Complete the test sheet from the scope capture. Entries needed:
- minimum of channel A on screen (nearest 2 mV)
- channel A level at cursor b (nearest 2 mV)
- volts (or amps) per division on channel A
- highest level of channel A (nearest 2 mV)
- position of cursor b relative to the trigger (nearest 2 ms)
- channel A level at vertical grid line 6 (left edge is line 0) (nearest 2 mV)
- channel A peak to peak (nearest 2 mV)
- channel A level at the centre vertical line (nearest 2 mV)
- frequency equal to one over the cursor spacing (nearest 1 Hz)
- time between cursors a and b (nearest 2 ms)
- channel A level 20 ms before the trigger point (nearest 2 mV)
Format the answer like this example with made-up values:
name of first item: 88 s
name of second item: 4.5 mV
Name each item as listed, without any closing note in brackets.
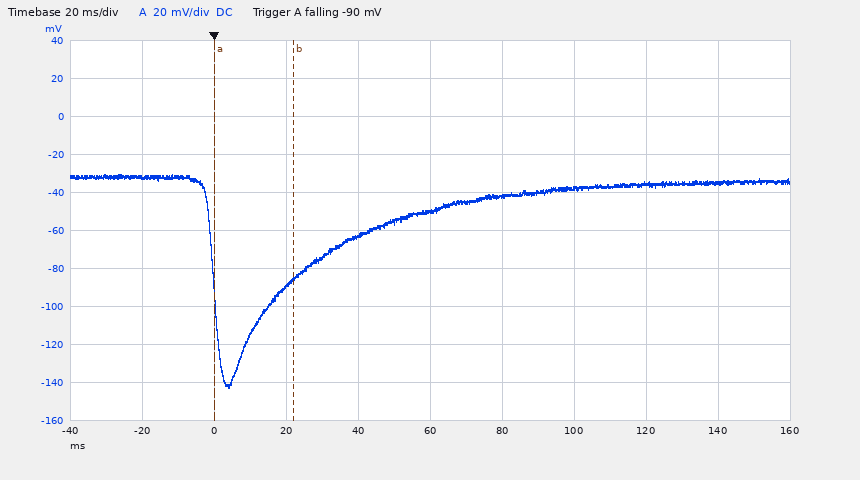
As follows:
minimum of channel A on screen: -142 mV
channel A level at cursor b: -86 mV
volts (or amps) per division on channel A: 20 mV
highest level of channel A: -30 mV
position of cursor b relative to the trigger: +22 ms
channel A level at vertical grid line 6 (left edge is line 0): -42 mV
channel A peak to peak: 112 mV
channel A level at the centre vertical line: -50 mV
frequency equal to one over the cursor spacing: 45 Hz
time between cursors a and b: 22 ms
channel A level 20 ms before the trigger point: -32 mV
